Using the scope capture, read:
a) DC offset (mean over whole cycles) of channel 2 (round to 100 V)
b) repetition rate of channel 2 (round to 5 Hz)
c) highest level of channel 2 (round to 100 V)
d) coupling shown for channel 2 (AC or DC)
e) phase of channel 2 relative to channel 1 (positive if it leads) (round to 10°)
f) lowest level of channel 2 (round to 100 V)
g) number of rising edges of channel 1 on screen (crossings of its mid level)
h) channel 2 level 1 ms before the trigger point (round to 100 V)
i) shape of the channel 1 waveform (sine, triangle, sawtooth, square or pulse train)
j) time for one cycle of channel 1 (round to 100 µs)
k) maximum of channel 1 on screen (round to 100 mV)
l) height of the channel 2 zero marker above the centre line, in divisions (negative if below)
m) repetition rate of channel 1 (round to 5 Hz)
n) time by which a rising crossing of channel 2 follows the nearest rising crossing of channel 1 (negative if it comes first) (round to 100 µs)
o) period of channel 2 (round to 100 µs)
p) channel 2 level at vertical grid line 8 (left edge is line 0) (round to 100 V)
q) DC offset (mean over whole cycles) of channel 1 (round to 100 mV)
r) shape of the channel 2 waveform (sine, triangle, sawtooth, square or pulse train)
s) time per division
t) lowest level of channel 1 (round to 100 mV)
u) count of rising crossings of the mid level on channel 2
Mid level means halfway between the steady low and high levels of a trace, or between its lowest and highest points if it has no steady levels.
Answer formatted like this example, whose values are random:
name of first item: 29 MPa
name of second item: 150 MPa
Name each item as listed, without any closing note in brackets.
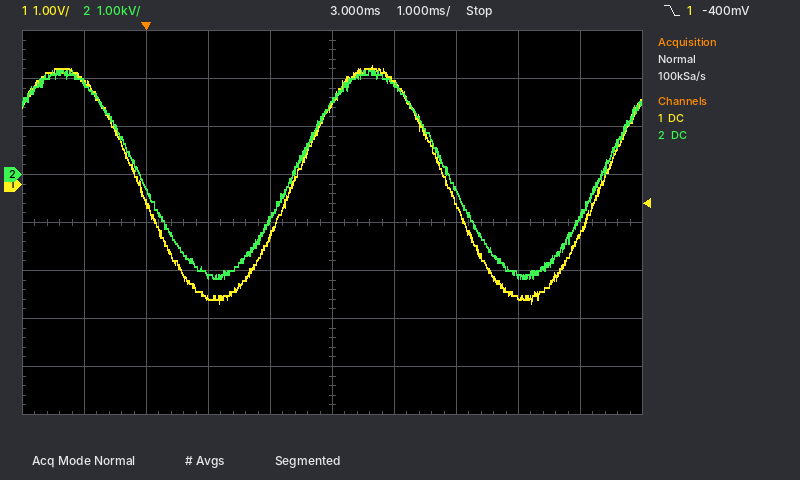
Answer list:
DC offset (mean over whole cycles) of channel 2: 0.0 kV
repetition rate of channel 2: 200 Hz
highest level of channel 2: 2.2 kV
coupling shown for channel 2: DC
phase of channel 2 relative to channel 1 (positive if it leads): 0°
lowest level of channel 2: -2.2 kV
number of rising edges of channel 1 on screen: 2
channel 2 level 1 ms before the trigger point: 1.9 kV
shape of the channel 1 waveform: sine
time for one cycle of channel 1: 5.0 ms
maximum of channel 1 on screen: 2.5 V
height of the channel 2 zero marker above the centre line, in divisions: +1.0 div
repetition rate of channel 1: 200 Hz
time by which a rising crossing of channel 2 follows the nearest rising crossing of channel 1 (negative if it comes first): 0.0 ms
period of channel 2: 5.0 ms
channel 2 level at vertical grid line 8 (left edge is line 0): -2.1 kV
DC offset (mean over whole cycles) of channel 1: 0.0 V
shape of the channel 2 waveform: sine
time per division: 1 ms
lowest level of channel 1: -2.5 V
count of rising crossings of the mid level on channel 2: 2
